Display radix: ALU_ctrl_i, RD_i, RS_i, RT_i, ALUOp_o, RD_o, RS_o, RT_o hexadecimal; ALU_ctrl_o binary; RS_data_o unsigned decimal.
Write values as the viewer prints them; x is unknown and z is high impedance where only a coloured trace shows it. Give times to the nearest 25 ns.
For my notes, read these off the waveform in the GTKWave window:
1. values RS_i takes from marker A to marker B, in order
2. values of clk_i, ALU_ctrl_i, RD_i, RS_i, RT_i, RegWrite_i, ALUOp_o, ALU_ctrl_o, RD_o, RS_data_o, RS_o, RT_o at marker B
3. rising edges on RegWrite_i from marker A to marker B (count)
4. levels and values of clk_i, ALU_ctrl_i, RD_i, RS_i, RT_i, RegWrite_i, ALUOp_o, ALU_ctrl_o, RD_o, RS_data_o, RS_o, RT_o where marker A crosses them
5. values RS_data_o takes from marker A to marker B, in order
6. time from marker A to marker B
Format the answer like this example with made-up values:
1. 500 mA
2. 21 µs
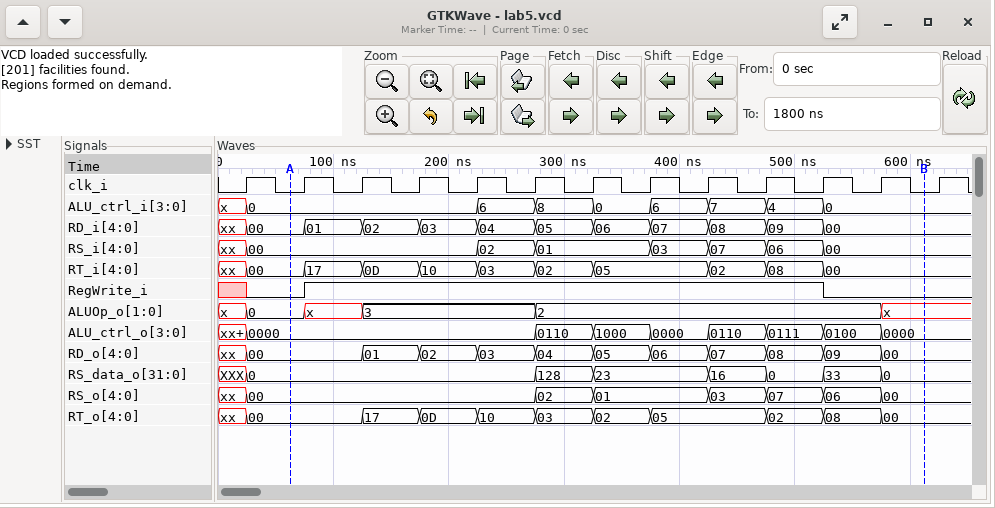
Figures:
1. 00, 02, 01, 03, 07, 06, 00
2. clk_i=0, ALU_ctrl_i=0, RD_i=00, RS_i=00, RT_i=00, RegWrite_i=0, ALUOp_o=x, ALU_ctrl_o=0000, RD_o=00, RS_data_o=0, RS_o=00, RT_o=00
3. 1
4. clk_i=0, ALU_ctrl_i=0, RD_i=00, RS_i=00, RT_i=00, RegWrite_i=0, ALUOp_o=0, ALU_ctrl_o=0000, RD_o=00, RS_data_o=0, RS_o=00, RT_o=00
5. 0, 128, 23, 16, 0, 33, 0
6. 550 ns
